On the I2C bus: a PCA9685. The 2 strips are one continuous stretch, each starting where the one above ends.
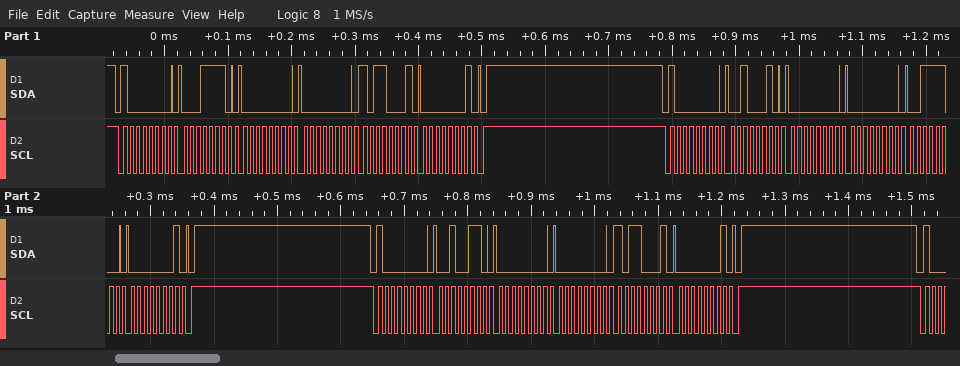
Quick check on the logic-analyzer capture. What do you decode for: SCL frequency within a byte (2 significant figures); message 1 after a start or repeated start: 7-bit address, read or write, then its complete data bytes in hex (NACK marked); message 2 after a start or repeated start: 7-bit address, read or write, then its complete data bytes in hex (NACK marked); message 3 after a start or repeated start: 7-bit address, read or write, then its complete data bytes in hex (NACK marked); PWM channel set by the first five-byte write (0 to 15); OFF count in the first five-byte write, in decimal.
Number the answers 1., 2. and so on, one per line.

1. 100 kHz
2. 0x40 write: 1E 00 00 B1 01
3. 0x40 write: 22 00 00 3C 01
4. 0x40 write: 26 00 00 B1 01
5. 6
6. 433
